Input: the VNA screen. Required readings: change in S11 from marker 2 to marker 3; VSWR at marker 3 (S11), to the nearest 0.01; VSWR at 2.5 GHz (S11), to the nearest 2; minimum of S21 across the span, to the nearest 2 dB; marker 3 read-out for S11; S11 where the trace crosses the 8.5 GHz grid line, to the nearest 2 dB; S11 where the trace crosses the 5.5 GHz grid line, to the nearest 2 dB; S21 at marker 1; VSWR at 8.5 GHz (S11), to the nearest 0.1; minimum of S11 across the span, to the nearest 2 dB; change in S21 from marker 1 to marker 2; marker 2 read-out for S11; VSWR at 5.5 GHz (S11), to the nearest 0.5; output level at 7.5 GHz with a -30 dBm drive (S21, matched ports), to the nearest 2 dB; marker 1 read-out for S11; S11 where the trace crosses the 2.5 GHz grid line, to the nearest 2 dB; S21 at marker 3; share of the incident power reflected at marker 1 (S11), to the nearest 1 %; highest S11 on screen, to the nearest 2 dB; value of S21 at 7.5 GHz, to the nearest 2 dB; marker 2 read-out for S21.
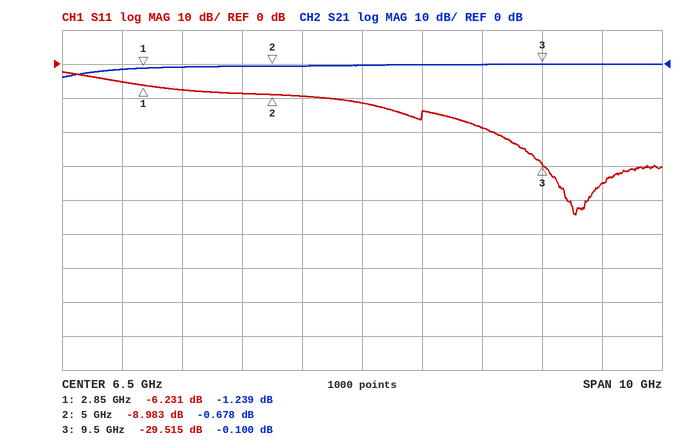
-20.532 dB
1.07
4
-4 dB
-29.515 dB
-18 dB
-10 dB
-1.239 dB
1.3
-44 dB
0.561 dB
-8.983 dB
2.0
-30 dBm
-6.231 dB
-6 dB
-0.100 dB
24 %
-2 dB
0 dB
-0.678 dB
